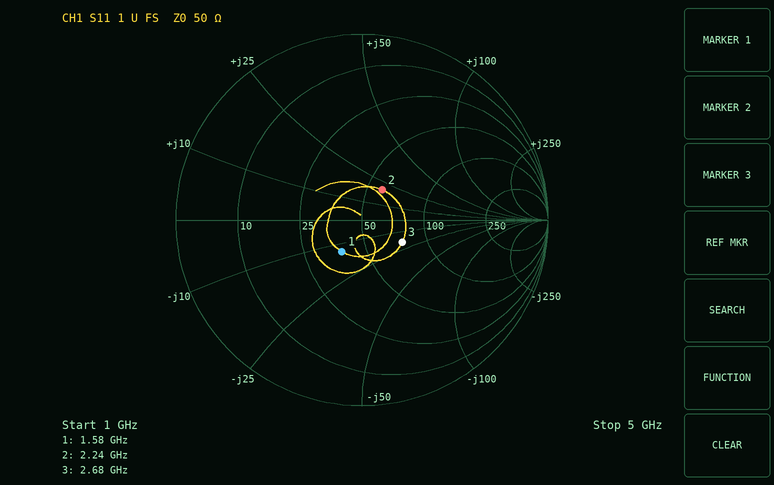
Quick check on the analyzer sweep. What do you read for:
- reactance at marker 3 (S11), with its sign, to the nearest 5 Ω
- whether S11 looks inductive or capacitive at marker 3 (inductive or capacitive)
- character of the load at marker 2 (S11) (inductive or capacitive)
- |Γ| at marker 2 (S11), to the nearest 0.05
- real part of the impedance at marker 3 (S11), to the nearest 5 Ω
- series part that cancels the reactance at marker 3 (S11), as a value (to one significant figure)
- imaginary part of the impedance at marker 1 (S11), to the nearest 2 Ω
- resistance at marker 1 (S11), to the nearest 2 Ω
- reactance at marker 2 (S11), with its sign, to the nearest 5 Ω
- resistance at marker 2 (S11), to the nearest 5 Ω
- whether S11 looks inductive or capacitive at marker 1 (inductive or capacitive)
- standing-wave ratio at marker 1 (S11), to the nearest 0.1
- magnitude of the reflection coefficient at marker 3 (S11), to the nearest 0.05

-20 Ω
capacitive
inductive
0.20
75 Ω
1 nH
-14 Ω
38 Ω
+20 Ω
60 Ω
capacitive
1.5
0.25
